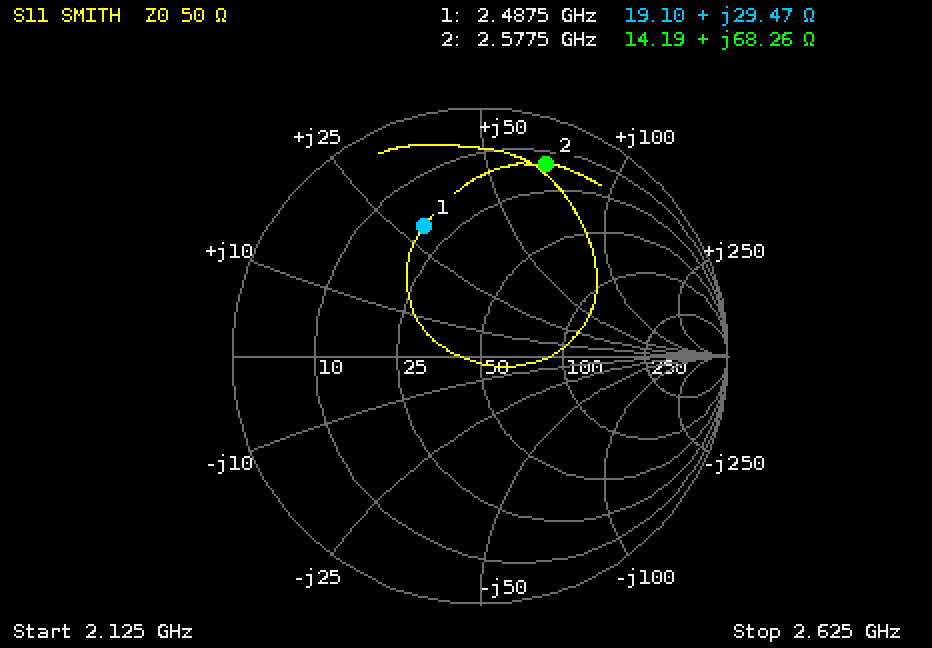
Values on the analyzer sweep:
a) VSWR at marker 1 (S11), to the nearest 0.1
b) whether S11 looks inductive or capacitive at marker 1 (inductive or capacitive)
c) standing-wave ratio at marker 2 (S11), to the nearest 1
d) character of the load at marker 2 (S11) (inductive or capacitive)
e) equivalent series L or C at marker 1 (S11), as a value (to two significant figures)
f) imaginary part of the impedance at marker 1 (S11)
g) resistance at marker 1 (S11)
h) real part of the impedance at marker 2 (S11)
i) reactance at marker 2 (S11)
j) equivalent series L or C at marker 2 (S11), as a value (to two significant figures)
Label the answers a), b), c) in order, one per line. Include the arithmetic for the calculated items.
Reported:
a) 3.6
b) inductive
c) 10
d) inductive
e) L = 29.47 Ω/(2π × 2.4875 GHz) ≈ 1.9 nH
f) +29.47 Ω
g) 19.10 Ω
h) 14.19 Ω
i) +68.26 Ω
j) L = 68.26 Ω/(2π × 2.5775 GHz) ≈ 4.2 nH
